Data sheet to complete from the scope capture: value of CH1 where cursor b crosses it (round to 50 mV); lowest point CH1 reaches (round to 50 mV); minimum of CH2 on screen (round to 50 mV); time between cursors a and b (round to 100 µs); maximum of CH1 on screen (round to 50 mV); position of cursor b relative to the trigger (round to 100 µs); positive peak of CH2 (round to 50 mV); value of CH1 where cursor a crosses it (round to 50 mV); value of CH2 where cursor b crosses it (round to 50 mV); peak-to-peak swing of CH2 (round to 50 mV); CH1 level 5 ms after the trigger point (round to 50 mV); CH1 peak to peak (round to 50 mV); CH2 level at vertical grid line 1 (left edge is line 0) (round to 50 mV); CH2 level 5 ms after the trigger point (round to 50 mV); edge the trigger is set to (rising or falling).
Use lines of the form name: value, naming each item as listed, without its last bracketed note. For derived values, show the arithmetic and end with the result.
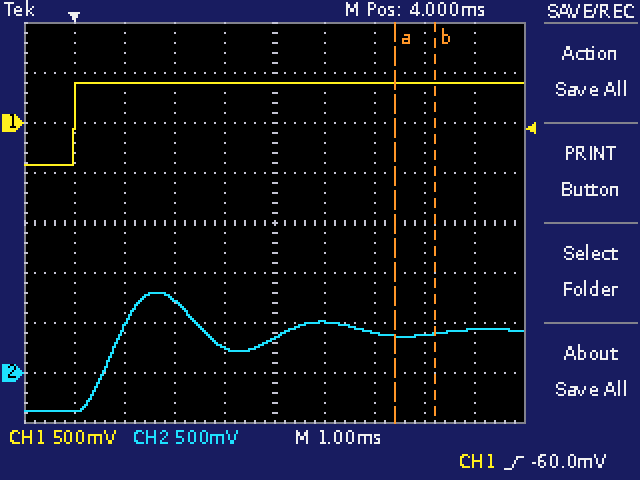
value of CH1 where cursor b crosses it: 400 mV
lowest point CH1 reaches: -400 mV
minimum of CH2 on screen: -400 mV
time between cursors a and b: 800 µs
maximum of CH1 on screen: 400 mV
position of cursor b relative to the trigger: +7.2 ms
positive peak of CH2: 800 mV
value of CH1 where cursor a crosses it: 400 mV
value of CH2 where cursor b crosses it: 400 mV
peak-to-peak swing of CH2: 800 mV − (-400 mV) = 1.20 V
CH1 level 5 ms after the trigger point: 400 mV
CH1 peak to peak: 400 mV − (-400 mV) = 800 mV
CH2 level at vertical grid line 1 (left edge is line 0): -400 mV
CH2 level 5 ms after the trigger point: 500 mV
edge the trigger is set to: rising
